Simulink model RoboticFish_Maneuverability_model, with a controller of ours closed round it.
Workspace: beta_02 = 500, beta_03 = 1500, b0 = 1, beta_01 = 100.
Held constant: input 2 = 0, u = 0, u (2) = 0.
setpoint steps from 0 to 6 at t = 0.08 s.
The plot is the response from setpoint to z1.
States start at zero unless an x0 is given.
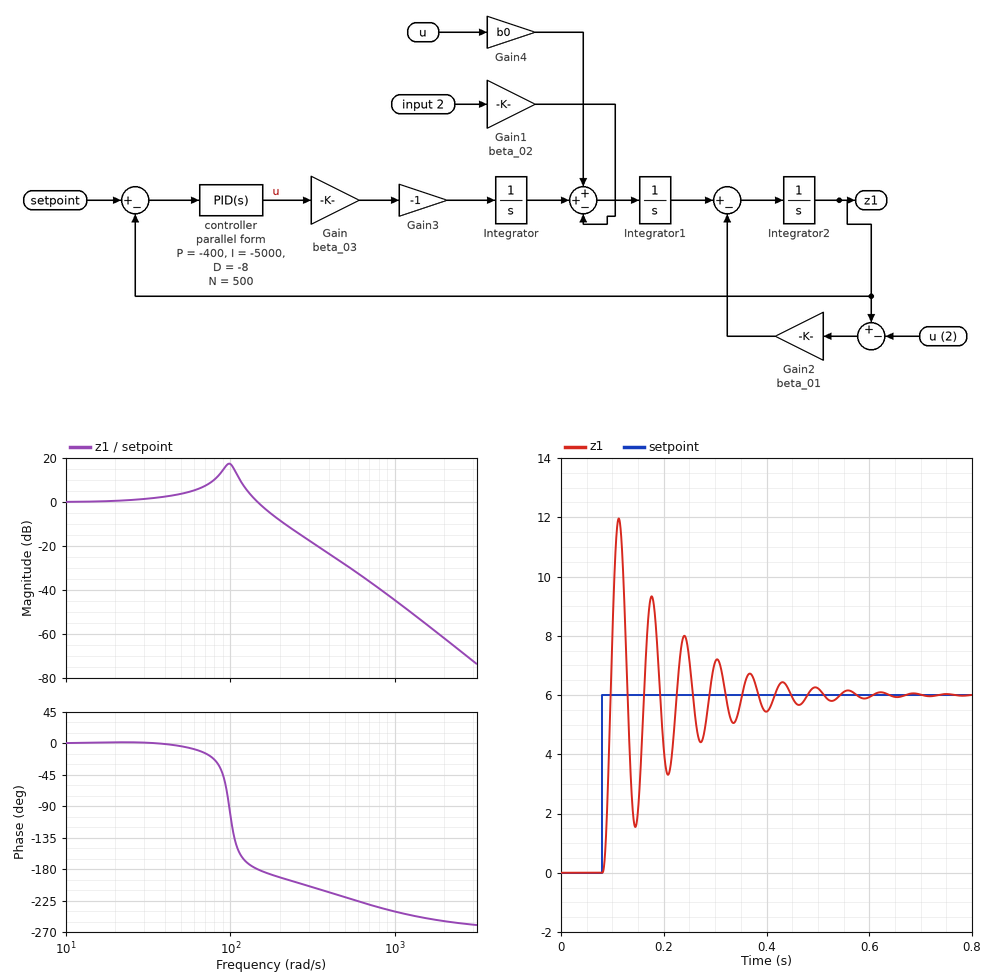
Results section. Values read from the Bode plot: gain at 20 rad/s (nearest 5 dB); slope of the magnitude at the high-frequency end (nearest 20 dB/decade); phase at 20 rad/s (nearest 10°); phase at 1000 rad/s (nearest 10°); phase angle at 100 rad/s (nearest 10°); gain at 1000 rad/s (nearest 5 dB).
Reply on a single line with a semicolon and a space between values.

0 dB; -60 dB/decade; 0°; -240°; -100°; -45 dB
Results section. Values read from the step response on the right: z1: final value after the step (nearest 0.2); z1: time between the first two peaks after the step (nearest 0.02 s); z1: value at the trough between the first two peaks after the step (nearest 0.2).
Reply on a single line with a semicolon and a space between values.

6.0; 0.06 s; 1.6
